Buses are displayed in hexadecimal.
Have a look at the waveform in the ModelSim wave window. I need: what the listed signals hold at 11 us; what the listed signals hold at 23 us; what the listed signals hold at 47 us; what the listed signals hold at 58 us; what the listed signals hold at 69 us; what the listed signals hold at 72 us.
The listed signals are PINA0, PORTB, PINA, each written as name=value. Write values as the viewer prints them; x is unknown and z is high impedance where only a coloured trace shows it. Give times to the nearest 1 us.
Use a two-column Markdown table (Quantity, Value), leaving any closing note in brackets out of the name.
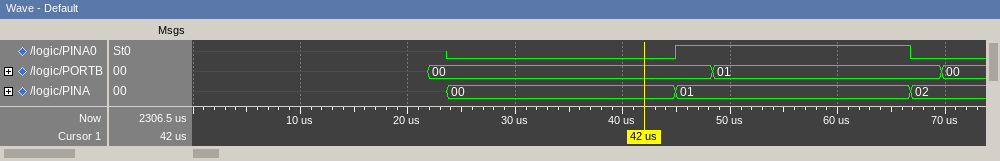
| Quantity | Value |
|---|---|
| what the listed signals hold at 11 us | PINA0=x, PORTB=x, PINA=x |
| what the listed signals hold at 23 us | PINA0=x, PORTB=00, PINA=x |
| what the listed signals hold at 47 us | PINA0=1, PORTB=00, PINA=01 |
| what the listed signals hold at 58 us | PINA0=1, PORTB=01, PINA=01 |
| what the listed signals hold at 69 us | PINA0=0, PORTB=01, PINA=02 |
| what the listed signals hold at 72 us | PINA0=0, PORTB=00, PINA=02 |
